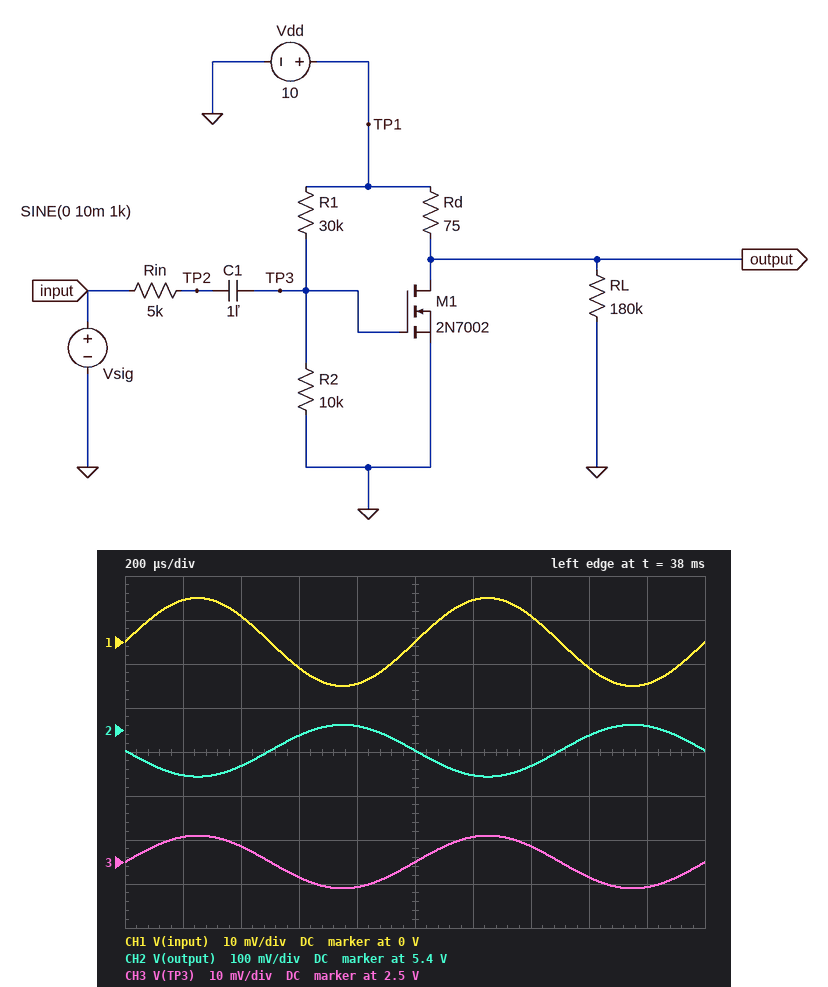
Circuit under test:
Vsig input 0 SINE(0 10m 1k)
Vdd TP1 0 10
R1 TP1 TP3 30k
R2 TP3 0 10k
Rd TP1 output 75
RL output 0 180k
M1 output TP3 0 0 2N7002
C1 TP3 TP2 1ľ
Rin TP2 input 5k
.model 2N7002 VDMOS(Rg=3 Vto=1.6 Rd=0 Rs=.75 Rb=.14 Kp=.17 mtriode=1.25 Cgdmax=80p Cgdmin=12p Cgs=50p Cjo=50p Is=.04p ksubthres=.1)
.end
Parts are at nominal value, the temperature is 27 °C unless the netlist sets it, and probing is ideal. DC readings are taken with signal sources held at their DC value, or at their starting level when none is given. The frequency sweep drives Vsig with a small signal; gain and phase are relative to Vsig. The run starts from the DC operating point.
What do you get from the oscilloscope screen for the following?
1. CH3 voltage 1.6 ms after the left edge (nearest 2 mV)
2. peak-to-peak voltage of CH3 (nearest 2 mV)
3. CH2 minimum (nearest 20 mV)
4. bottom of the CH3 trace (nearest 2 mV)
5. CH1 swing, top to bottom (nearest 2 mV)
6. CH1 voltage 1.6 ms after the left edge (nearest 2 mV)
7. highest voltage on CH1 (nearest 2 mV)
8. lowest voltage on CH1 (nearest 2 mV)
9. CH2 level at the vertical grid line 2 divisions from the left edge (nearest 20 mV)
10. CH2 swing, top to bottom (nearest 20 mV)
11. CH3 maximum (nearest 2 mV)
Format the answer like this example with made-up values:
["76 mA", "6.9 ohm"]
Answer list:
["2.496 V", "12 mV", "5.30 V", "2.494 V", "20 mV", "-6 mV", "10 mV", "-10 mV", "5.32 V", "120 mV", "2.506 V"]
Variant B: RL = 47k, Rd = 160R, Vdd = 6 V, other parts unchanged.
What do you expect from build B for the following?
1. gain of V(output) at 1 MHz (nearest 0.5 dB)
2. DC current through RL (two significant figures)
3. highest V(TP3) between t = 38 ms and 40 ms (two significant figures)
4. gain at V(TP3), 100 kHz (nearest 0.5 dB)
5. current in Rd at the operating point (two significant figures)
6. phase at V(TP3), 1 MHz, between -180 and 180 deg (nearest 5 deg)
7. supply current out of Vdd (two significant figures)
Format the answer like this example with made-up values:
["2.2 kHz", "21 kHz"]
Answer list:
["-22.0 dB", "130 µA", "1.5 V", "-4.5 dB", "210 µA", "-55 deg", "360 µA"]
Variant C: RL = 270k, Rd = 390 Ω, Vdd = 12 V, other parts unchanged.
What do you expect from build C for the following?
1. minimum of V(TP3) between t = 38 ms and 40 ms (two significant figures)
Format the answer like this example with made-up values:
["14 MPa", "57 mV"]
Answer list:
["3.0 V"]
